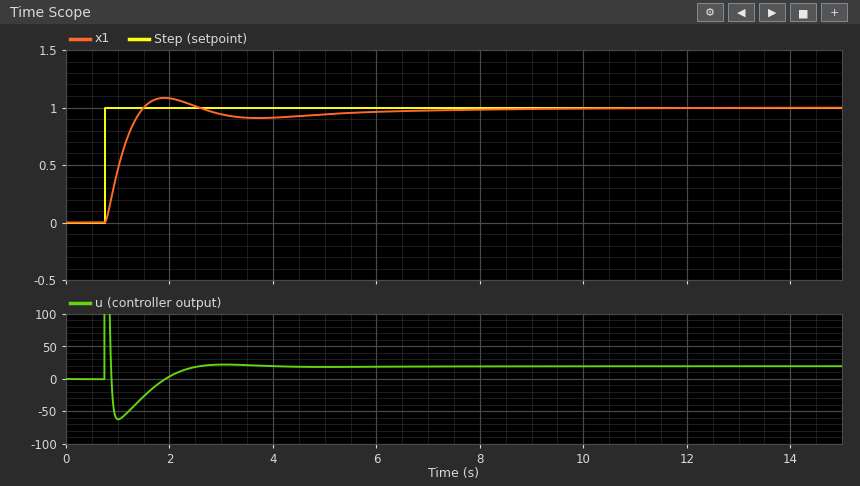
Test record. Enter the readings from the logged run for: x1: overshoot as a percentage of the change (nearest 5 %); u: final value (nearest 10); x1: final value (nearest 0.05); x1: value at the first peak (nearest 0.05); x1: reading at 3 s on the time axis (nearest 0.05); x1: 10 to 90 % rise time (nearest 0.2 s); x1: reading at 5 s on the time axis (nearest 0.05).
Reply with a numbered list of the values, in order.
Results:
1. 10 %
2. 20
3. 1.00
4. 1.10
5. 0.95
6. 0.6 s
7. 0.95
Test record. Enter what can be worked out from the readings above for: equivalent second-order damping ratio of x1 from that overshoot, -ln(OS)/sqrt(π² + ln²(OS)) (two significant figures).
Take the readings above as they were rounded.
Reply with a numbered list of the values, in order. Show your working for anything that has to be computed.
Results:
1. ln(0.1) = -2.303; 2.303 / sqrt(9.870 + 5.302) = 0.59
